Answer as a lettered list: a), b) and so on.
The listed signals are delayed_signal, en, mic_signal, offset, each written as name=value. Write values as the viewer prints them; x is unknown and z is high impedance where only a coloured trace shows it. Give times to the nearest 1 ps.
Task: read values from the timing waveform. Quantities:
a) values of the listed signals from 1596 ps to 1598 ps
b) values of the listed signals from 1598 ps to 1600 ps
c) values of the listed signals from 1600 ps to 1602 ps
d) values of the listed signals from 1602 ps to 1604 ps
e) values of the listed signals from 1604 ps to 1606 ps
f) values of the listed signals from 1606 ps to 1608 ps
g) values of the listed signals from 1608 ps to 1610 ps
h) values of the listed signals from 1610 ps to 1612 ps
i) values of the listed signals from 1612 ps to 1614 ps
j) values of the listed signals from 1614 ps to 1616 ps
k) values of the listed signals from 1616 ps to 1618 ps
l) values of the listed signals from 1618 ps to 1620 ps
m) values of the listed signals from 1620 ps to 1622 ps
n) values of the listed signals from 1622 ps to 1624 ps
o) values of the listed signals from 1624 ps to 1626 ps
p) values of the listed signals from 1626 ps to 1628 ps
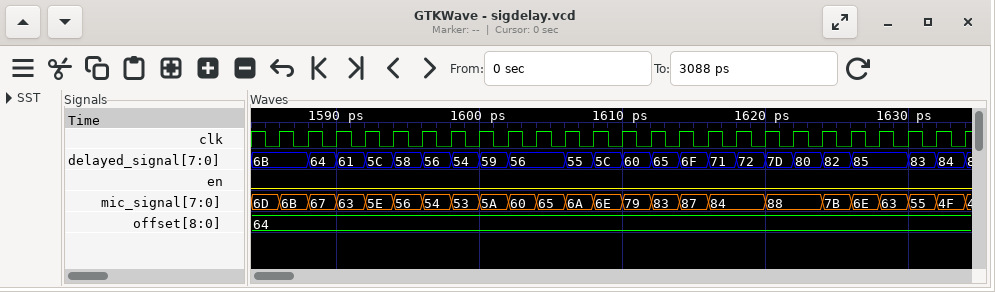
a) delayed_signal=56, en=0, mic_signal=54, offset=64
b) delayed_signal=54, en=0, mic_signal=53, offset=64
c) delayed_signal=59, en=0, mic_signal=5A, offset=64
d) delayed_signal=56, en=0, mic_signal=60, offset=64
e) delayed_signal=56, en=0, mic_signal=65, offset=64
f) delayed_signal=55, en=0, mic_signal=6A, offset=64
g) delayed_signal=5C, en=0, mic_signal=6E, offset=64
h) delayed_signal=60, en=0, mic_signal=79, offset=64
i) delayed_signal=65, en=0, mic_signal=83, offset=64
j) delayed_signal=6F, en=0, mic_signal=87, offset=64
k) delayed_signal=71, en=0, mic_signal=84, offset=64
l) delayed_signal=72, en=0, mic_signal=84, offset=64
m) delayed_signal=7D, en=0, mic_signal=88, offset=64
n) delayed_signal=80, en=0, mic_signal=88, offset=64
o) delayed_signal=82, en=0, mic_signal=7B, offset=64
p) delayed_signal=85, en=0, mic_signal=6E, offset=64
